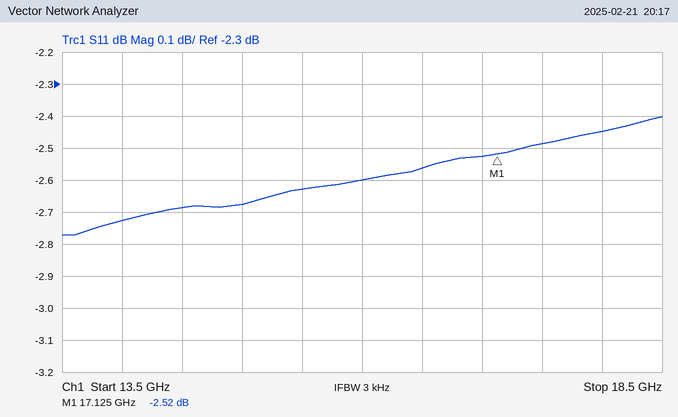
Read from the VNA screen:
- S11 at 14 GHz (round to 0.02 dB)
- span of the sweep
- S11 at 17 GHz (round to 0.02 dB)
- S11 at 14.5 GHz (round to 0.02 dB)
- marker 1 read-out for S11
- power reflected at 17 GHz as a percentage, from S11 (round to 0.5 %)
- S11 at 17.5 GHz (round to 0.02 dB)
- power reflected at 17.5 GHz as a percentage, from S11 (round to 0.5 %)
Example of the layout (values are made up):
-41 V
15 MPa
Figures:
-2.72 dB
5 GHz
-2.52 dB
-2.68 dB
-2.52 dB
56.0 %
-2.48 dB
56.5 %
